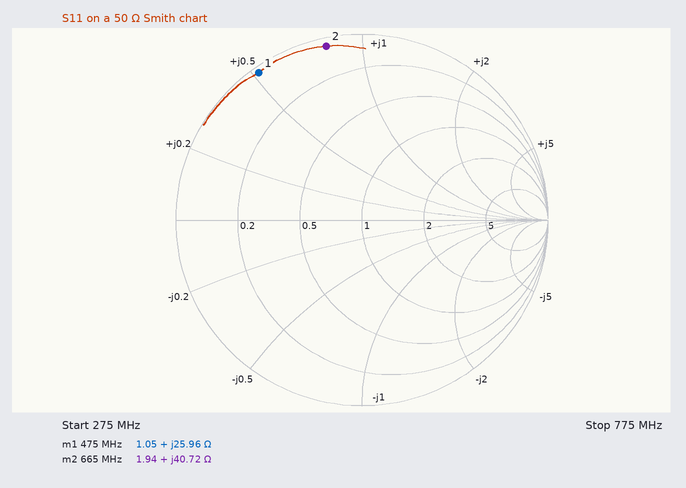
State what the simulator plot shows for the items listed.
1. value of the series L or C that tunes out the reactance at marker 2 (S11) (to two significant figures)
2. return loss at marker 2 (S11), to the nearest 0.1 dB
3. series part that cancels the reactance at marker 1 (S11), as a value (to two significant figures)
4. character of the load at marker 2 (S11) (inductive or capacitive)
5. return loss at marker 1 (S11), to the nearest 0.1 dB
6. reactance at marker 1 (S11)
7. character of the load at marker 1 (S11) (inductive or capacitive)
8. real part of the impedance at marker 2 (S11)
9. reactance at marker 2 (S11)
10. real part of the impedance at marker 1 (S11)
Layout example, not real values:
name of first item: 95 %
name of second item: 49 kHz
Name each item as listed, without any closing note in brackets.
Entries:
value of the series L or C that tunes out the reactance at marker 2 (S11): 5.9 pF
return loss at marker 2 (S11), to the nearest 0.1 dB: 0.4 dB
series part that cancels the reactance at marker 1 (S11), as a value: 13 pF
character of the load at marker 2 (S11): inductive
return loss at marker 1 (S11), to the nearest 0.1 dB: 0.3 dB
reactance at marker 1: +25.96 Ω
character of the load at marker 1 (S11): inductive
real part of the impedance at marker 2: 1.94 Ω
reactance at marker 2: +40.72 Ω
real part of the impedance at marker 1: 1.05 Ω
